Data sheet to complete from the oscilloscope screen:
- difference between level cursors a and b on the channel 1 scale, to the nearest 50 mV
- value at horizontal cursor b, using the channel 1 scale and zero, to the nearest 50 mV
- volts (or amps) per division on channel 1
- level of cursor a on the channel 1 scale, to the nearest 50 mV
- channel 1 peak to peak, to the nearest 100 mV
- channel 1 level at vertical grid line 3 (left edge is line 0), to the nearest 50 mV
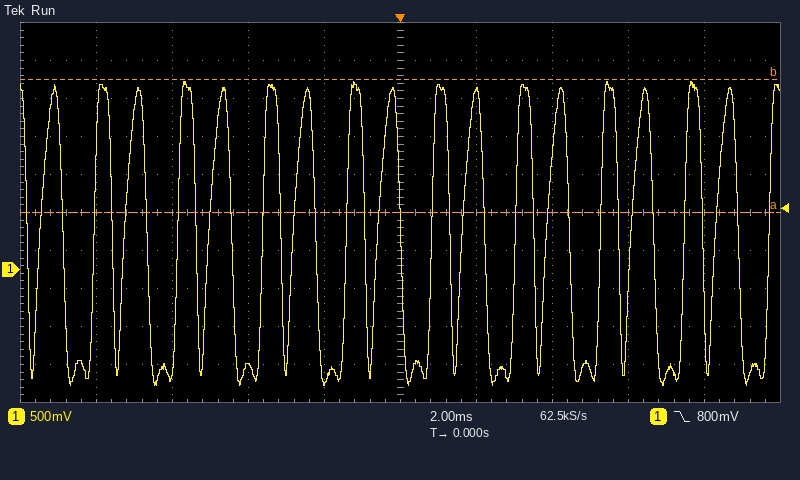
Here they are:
1.75 V
2.50 V
500 mV
750 mV
4.00 V
-1.30 V
